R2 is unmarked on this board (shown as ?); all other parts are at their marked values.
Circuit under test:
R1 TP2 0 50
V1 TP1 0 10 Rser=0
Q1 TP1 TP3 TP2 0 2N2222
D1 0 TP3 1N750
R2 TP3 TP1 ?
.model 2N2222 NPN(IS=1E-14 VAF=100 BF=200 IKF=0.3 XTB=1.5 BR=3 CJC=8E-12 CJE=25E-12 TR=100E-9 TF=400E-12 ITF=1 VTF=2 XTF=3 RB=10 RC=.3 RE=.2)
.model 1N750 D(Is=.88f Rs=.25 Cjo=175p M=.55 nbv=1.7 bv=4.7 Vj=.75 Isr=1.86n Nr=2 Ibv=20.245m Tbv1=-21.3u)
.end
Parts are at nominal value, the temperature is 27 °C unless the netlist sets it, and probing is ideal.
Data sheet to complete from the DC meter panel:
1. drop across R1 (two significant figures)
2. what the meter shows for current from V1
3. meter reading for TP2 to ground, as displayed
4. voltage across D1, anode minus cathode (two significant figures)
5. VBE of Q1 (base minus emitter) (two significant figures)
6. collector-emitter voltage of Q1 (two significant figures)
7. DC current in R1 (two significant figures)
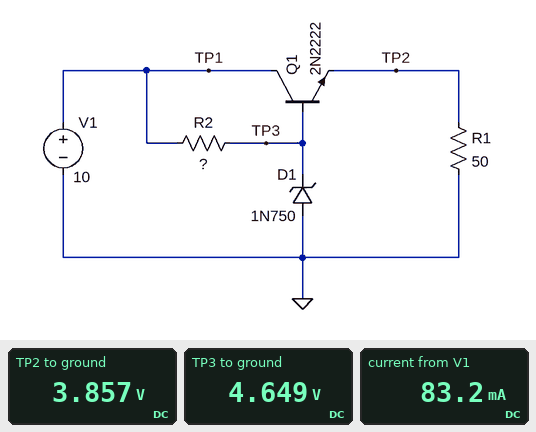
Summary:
3.9 V
83.2 mA
3.857 V
-4.6 V
790 mV
6.1 V
77 mA
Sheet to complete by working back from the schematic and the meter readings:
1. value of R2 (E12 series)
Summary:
820 Ω
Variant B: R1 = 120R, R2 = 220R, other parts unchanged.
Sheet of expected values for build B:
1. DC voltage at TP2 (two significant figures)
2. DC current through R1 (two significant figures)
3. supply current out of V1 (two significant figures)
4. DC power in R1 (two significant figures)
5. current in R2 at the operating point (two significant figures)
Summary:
4.0 V
33 mA
57 mA
130 mW
24 mA
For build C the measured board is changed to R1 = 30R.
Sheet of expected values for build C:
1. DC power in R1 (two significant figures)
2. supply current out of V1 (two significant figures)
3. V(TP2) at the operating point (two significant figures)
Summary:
490 mW
130 mA
3.8 V
